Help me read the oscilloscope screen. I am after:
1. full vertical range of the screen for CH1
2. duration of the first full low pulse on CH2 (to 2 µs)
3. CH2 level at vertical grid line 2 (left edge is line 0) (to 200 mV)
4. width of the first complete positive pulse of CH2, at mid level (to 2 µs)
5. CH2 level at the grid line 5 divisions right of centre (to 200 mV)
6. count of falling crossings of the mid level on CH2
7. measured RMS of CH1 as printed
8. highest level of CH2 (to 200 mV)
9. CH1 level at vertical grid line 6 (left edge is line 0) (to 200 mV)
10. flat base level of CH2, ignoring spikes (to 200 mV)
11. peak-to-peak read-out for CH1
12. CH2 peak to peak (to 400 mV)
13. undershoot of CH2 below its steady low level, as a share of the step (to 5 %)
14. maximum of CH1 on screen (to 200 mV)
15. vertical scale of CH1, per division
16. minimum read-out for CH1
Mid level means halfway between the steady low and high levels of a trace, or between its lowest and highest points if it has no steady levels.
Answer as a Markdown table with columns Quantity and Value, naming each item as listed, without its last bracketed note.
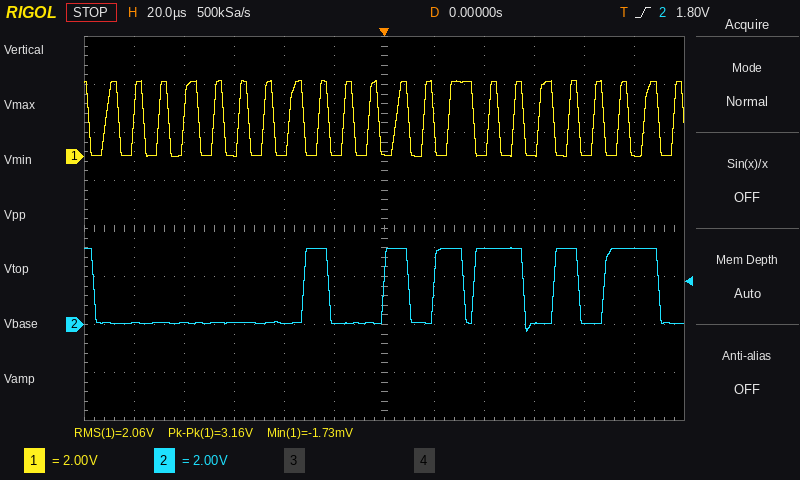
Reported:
| Quantity | Value |
|---|---|
| full vertical range of the screen for CH1 | 16 V |
| duration of the first full low pulse on CH2 | 84 µs |
| CH2 level at vertical grid line 2 (left edge is line 0) | 0.0 V |
| width of the first complete positive pulse of CH2, at mid level | 10 µs |
| CH2 level at the grid line 5 divisions right of centre | 3.2 V |
| count of falling crossings of the mid level on CH2 | 7 |
| measured RMS of CH1 as printed | 2.06 V |
| highest level of CH2 | 3.2 V |
| CH1 level at vertical grid line 6 (left edge is line 0) | 200 mV |
| flat base level of CH2, ignoring spikes | 0.0 V |
| peak-to-peak read-out for CH1 | 3.16 V |
| CH2 peak to peak | 3.6 V |
| undershoot of CH2 below its steady low level, as a share of the step | 10 % |
| maximum of CH1 on screen | 3.2 V |
| vertical scale of CH1, per division | 2 V |
| minimum read-out for CH1 | -1.73 mV |
